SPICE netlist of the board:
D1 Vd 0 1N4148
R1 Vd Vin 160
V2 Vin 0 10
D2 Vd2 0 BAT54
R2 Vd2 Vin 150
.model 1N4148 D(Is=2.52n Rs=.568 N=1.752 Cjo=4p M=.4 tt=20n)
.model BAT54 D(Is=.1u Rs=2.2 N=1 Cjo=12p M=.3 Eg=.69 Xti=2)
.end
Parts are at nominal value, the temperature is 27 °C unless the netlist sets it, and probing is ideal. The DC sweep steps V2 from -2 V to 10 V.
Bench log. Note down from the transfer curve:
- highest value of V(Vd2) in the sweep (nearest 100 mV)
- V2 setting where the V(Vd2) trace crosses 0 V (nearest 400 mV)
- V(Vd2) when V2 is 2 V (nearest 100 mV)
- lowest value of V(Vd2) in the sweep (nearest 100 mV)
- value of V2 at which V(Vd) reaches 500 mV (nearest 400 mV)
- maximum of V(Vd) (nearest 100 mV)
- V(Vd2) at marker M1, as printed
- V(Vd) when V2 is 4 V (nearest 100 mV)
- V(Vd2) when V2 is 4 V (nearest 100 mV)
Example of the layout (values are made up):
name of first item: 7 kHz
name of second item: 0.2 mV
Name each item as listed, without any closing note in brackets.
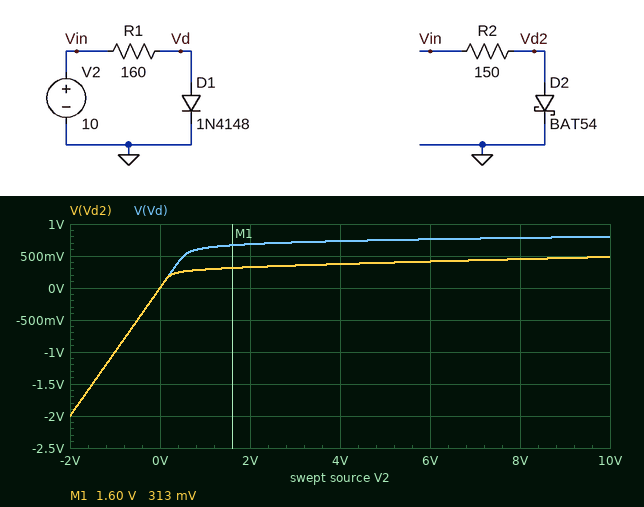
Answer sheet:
highest value of V(Vd2) in the sweep: 500 mV
V2 setting where the V(Vd2) trace crosses 0 V: 0 V
V(Vd2) when V2 is 2 V: 300 mV
lowest value of V(Vd2) in the sweep: -2.0 V
value of V2 at which V(Vd) reaches 500 mV: 400 mV
maximum of V(Vd): 800 mV
V(Vd2) at marker M1, as printed: 313 mV
V(Vd) when V2 is 4 V: 700 mV
V(Vd2) when V2 is 4 V: 400 mV
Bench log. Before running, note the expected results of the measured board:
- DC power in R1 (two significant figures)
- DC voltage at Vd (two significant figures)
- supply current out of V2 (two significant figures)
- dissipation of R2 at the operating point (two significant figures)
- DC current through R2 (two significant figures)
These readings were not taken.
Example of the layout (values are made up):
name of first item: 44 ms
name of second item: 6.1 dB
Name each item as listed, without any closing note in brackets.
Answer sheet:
DC power in R1: 530 mW
DC voltage at Vd: 800 mV
supply current out of V2: 120 mA
dissipation of R2 at the operating point: 600 mW
DC current through R2: 63 mA
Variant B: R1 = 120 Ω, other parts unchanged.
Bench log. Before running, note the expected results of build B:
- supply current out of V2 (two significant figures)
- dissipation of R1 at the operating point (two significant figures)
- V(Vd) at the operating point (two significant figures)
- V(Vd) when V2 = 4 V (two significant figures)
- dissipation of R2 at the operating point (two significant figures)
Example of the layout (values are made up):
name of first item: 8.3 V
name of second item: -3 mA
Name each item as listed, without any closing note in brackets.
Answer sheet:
supply current out of V2: 140 mA
dissipation of R1 at the operating point: 700 mW
V(Vd) at the operating point: 820 mV
V(Vd) when V2 = 4 V: 750 mV
dissipation of R2 at the operating point: 600 mW
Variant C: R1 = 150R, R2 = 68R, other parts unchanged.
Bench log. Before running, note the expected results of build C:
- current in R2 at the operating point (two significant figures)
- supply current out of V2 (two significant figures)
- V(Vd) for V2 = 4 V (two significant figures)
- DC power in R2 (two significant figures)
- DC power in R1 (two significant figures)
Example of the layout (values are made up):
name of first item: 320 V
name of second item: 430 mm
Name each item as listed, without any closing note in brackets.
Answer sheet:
current in R2 at the operating point: 140 mA
supply current out of V2: 200 mA
V(Vd) for V2 = 4 V: 740 mV
DC power in R2: 1.3 W
DC power in R1: 560 mW
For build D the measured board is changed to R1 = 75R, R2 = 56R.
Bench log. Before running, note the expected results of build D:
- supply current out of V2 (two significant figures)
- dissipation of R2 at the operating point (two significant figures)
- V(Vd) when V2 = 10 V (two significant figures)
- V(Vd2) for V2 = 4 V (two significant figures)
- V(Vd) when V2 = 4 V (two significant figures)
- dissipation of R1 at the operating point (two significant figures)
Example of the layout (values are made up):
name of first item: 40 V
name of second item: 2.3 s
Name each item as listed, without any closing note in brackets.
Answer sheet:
supply current out of V2: 290 mA
dissipation of R2 at the operating point: 1.5 W
V(Vd) when V2 = 10 V: 870 mV
V(Vd2) for V2 = 4 V: 480 mV
V(Vd) when V2 = 4 V: 780 mV
dissipation of R1 at the operating point: 1.1 W
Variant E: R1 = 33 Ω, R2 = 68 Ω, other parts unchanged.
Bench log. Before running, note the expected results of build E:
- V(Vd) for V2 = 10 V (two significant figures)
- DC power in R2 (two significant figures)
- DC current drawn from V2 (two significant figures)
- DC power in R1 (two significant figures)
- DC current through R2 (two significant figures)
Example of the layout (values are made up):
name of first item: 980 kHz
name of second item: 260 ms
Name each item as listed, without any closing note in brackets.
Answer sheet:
V(Vd) for V2 = 10 V: 990 mV
DC power in R2: 1.3 W
DC current drawn from V2: 410 mA
DC power in R1: 2.5 W
DC current through R2: 140 mA
